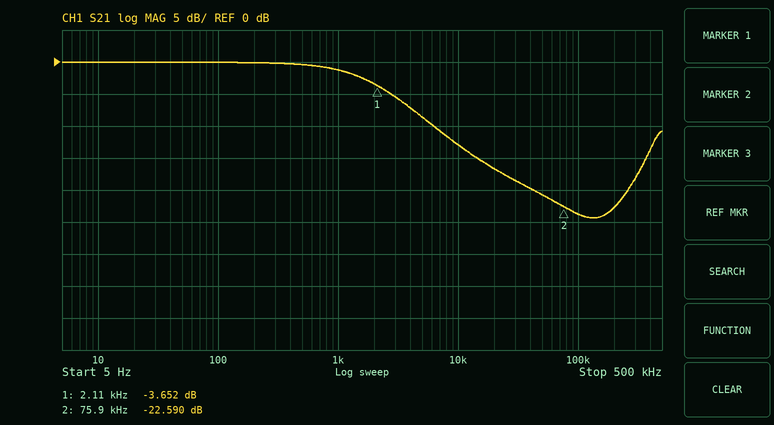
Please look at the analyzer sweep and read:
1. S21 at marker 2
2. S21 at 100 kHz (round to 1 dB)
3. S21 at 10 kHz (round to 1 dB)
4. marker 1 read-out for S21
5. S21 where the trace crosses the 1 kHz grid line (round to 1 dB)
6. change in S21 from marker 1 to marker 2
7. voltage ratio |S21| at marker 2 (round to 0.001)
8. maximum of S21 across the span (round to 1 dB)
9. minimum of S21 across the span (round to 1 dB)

-22.590 dB
-24 dB
-13 dB
-3.652 dB
-1 dB
-18.938 dB
0.074
0 dB
-24 dB
